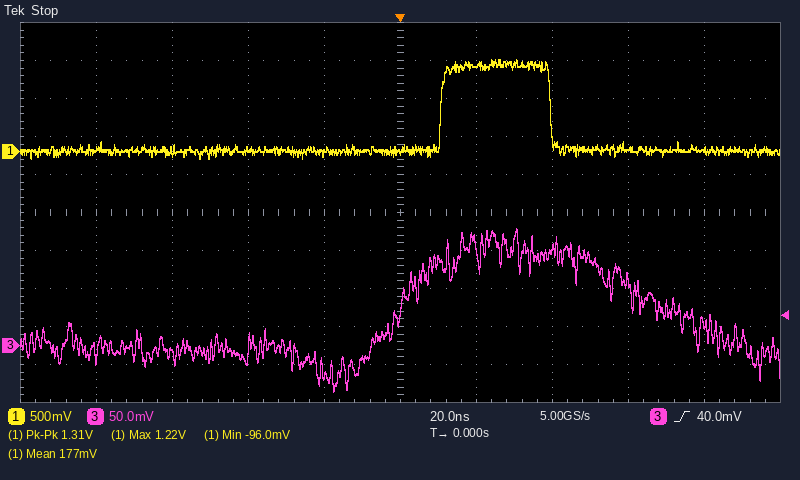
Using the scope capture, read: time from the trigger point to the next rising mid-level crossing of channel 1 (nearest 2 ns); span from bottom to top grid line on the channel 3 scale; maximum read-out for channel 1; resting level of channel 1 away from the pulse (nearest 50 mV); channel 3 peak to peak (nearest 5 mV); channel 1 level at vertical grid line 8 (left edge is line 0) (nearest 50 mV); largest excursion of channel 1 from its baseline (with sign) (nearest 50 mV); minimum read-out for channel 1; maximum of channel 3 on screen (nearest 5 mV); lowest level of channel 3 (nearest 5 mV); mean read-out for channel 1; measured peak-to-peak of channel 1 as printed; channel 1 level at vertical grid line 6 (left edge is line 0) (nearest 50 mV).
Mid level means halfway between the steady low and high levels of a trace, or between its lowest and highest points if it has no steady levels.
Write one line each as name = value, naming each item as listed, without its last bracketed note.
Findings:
time from the trigger point to the next rising mid-level crossing of channel 1 = 10 ns
span from bottom to top grid line on the channel 3 scale = 500 mV
maximum read-out for channel 1 = 1.22 V
resting level of channel 1 away from the pulse = 0 mV
channel 3 peak to peak = 215 mV
channel 1 level at vertical grid line 8 (left edge is line 0) = 50 mV
largest excursion of channel 1 from its baseline (with sign) = +1.20 V
minimum read-out for channel 1 = -96.0 mV
maximum of channel 3 on screen = 155 mV
lowest level of channel 3 = -60 mV
mean read-out for channel 1 = 177 mV
measured peak-to-peak of channel 1 as printed = 1.31 V
channel 1 level at vertical grid line 6 (left edge is line 0) = 1.15 V
